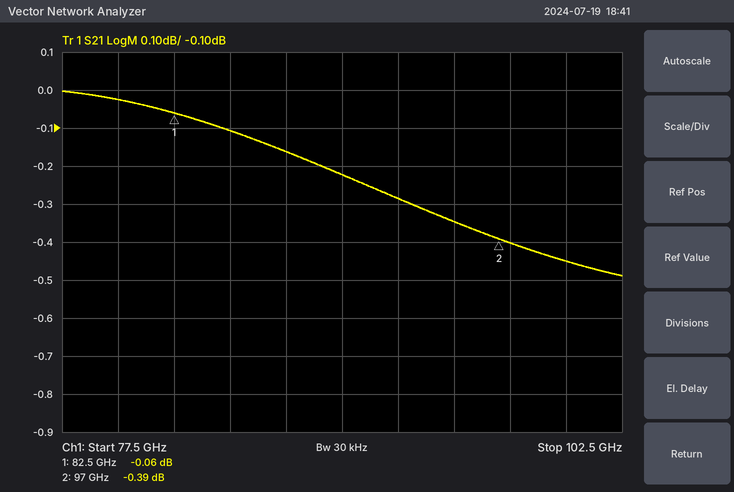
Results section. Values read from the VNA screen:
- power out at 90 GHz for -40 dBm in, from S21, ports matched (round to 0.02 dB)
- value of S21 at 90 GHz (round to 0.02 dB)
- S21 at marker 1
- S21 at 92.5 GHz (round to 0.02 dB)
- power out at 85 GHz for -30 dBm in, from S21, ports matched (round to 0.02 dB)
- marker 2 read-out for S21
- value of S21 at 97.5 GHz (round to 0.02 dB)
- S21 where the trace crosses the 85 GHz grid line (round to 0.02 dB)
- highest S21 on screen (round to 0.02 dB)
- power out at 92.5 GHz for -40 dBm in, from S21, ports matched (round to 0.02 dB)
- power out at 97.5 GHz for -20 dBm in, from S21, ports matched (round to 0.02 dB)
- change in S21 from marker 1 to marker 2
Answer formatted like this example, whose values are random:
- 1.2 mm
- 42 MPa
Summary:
- -40.22 dBm
- -0.22 dB
- -0.06 dB
- -0.28 dB
- -30.10 dBm
- -0.39 dB
- -0.40 dB
- -0.10 dB
- 0.00 dB
- -40.28 dBm
- -20.40 dBm
- -0.33 dB
